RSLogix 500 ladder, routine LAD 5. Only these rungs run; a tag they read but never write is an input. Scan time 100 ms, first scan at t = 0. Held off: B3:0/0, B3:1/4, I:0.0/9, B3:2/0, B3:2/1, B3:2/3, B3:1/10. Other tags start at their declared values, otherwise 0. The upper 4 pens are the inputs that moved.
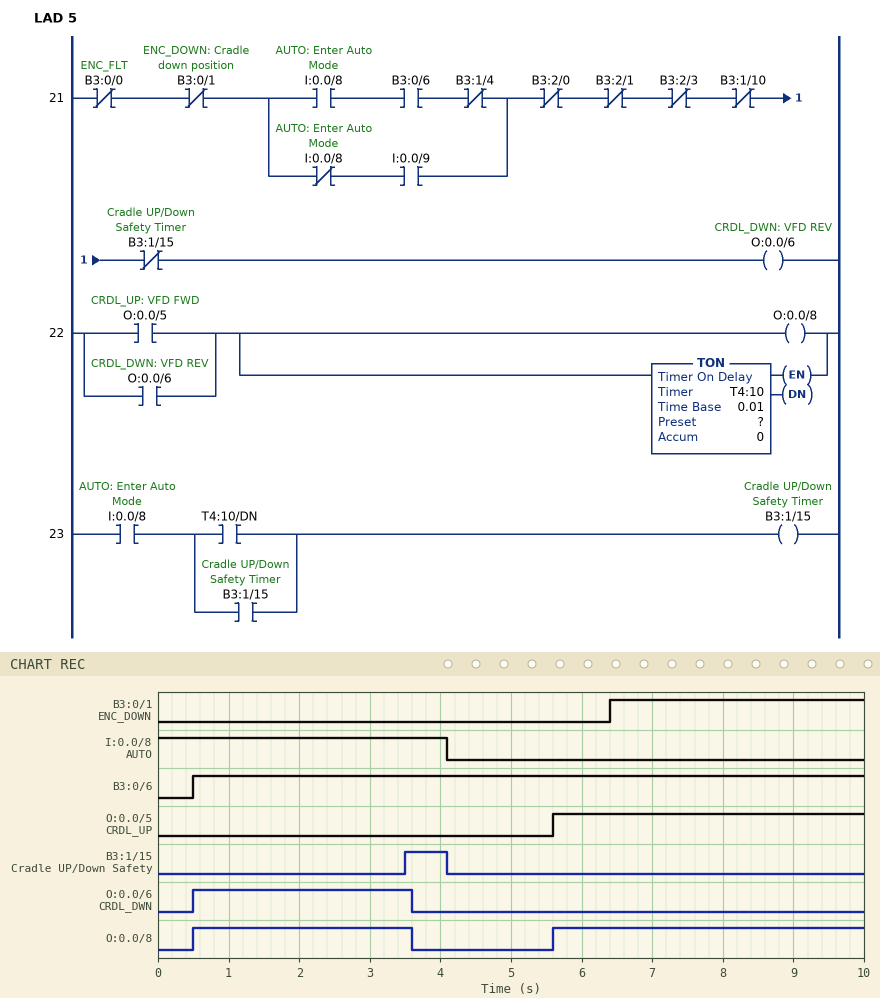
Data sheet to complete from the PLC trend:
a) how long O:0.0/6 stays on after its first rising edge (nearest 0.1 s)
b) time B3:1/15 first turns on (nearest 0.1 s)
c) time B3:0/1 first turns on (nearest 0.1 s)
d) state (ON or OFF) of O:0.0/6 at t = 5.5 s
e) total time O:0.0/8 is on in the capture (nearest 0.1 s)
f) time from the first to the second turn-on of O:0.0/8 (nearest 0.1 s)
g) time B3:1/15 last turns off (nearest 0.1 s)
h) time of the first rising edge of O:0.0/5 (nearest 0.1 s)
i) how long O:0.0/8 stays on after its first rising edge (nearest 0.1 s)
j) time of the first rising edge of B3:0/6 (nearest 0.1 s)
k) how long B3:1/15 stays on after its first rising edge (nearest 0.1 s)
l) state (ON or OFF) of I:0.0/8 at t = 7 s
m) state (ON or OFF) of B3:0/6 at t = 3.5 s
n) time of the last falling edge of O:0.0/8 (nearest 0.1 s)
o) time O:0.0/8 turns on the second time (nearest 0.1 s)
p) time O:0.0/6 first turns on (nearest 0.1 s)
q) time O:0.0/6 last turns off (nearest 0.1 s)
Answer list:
3.1 s
3.5 s
6.4 s
OFF
7.5 s
5.1 s
4.1 s
5.6 s
3.1 s
0.5 s
0.6 s
OFF
ON
3.6 s
5.6 s
0.5 s
3.6 s
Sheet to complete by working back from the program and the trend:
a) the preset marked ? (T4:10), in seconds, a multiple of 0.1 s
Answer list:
3.0 s
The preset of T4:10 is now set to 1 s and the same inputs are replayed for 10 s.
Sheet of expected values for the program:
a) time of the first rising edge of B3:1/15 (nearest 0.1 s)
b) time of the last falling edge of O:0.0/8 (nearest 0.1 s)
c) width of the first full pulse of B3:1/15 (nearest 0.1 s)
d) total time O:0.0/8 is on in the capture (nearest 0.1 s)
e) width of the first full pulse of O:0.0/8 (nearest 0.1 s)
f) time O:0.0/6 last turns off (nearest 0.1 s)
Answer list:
1.5 s
1.6 s
2.6 s
5.5 s
1.1 s
1.6 s
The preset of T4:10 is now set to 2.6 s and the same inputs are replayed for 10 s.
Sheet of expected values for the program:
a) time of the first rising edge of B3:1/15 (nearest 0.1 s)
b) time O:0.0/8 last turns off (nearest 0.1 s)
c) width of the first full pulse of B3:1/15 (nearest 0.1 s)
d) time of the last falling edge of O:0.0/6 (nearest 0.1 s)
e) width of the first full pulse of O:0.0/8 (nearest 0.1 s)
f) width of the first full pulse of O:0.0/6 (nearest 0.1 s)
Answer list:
3.1 s
3.2 s
1.0 s
3.2 s
2.7 s
2.7 s
